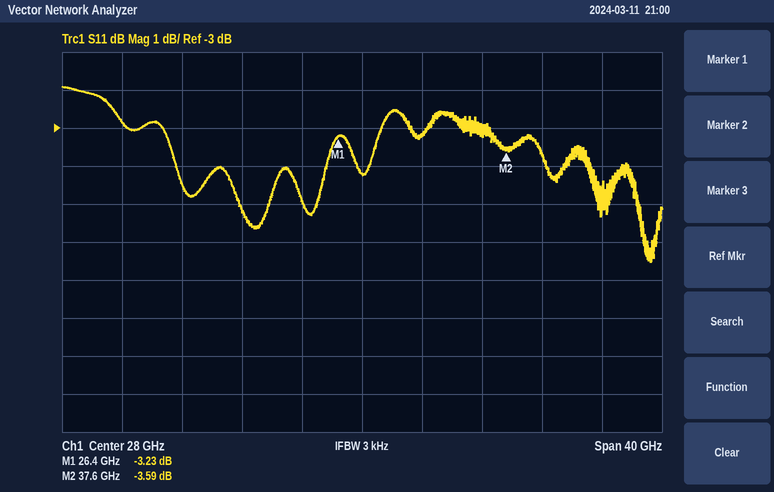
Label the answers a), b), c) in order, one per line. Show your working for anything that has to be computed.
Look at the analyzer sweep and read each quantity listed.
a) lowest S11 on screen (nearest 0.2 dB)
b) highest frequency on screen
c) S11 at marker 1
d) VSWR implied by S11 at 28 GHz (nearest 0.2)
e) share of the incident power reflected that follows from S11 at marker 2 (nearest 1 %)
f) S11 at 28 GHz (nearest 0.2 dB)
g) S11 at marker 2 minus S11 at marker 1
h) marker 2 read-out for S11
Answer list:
a) -6.6 dB
b) 48 GHz
c) -3.23 dB
d) |Γ| = 10^(-4.2/20) = 0.6166; VSWR = (1 + 0.6166)/(1 − 0.6166) ≈ 4.2
e) 10^(-3.59/10) ≈ 44 %
f) -4.2 dB
g) -3.59 − (-3.23) = -0.36 dB
h) -3.59 dB
